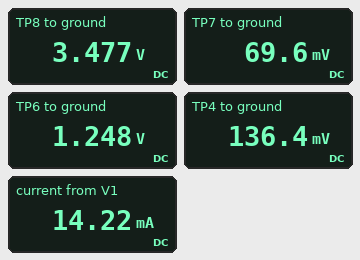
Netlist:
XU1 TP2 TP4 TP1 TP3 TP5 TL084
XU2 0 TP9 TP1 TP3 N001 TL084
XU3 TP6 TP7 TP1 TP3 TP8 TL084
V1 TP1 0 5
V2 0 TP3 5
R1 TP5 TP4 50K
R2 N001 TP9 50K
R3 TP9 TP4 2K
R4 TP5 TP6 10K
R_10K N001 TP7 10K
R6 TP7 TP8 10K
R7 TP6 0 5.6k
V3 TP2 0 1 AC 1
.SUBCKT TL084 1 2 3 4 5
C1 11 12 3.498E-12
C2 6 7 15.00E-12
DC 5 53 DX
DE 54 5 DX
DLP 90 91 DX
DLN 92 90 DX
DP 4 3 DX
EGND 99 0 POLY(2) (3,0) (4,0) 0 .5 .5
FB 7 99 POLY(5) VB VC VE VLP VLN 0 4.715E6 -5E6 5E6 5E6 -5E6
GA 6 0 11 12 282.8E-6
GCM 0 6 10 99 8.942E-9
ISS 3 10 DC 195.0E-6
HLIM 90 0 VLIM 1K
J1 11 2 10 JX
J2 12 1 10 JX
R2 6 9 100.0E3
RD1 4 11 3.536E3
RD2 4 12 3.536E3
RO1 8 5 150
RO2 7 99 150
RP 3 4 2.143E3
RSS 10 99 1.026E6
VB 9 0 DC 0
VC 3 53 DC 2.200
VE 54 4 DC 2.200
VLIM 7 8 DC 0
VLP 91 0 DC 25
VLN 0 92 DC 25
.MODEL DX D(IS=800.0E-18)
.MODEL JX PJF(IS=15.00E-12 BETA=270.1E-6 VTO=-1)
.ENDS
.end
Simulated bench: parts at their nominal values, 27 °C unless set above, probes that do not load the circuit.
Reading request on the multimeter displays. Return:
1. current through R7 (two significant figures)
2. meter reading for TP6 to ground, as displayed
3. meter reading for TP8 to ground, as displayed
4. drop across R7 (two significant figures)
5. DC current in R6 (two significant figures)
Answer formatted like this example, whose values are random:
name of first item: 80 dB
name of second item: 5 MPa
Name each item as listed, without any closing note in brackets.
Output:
current through R7: 220 µA
meter reading for TP6 to ground, as displayed: 1.248 V
meter reading for TP8 to ground, as displayed: 3.477 V
drop across R7: 1.2 V
DC current in R6: 340 µA
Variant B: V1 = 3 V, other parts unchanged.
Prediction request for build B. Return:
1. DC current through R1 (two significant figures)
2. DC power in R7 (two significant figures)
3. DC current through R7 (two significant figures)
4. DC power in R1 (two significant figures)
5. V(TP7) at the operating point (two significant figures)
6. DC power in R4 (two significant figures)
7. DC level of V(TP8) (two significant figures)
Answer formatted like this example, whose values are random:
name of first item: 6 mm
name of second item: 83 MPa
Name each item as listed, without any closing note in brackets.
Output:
DC current through R1: 28 µA
DC power in R7: 50 µW
DC current through R7: 95 µA
DC power in R1: 40 µW
V(TP7) at the operating point: 25 mV
DC power in R4: 90 µW
DC level of V(TP8): 1.5 V
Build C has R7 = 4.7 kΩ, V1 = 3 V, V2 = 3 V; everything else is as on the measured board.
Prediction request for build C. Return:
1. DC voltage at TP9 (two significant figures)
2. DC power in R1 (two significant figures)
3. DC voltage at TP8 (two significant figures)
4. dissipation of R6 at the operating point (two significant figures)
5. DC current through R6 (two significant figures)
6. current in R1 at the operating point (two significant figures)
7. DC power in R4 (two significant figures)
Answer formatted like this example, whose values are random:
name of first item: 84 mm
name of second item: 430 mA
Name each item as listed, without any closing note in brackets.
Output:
DC voltage at TP9: 18 mV
DC power in R1: 39 µW
DC voltage at TP8: 1.5 V
dissipation of R6 at the operating point: 200 µW
DC current through R6: 140 µA
current in R1 at the operating point: 28 µA
DC power in R4: 100 µW
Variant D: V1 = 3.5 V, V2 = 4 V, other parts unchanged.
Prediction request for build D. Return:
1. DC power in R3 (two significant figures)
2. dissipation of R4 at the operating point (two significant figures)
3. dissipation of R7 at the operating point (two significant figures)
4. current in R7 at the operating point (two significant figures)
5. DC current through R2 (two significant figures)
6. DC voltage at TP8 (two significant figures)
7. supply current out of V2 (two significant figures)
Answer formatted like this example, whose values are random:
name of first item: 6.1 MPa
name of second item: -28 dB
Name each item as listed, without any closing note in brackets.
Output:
DC power in R3: 2.9 µW
dissipation of R4 at the operating point: 160 µW
dissipation of R7 at the operating point: 90 µW
current in R7 at the operating point: 130 µA
DC current through R2: 38 µA
DC voltage at TP8: 2.0 V
supply current out of V2: 11 mA
